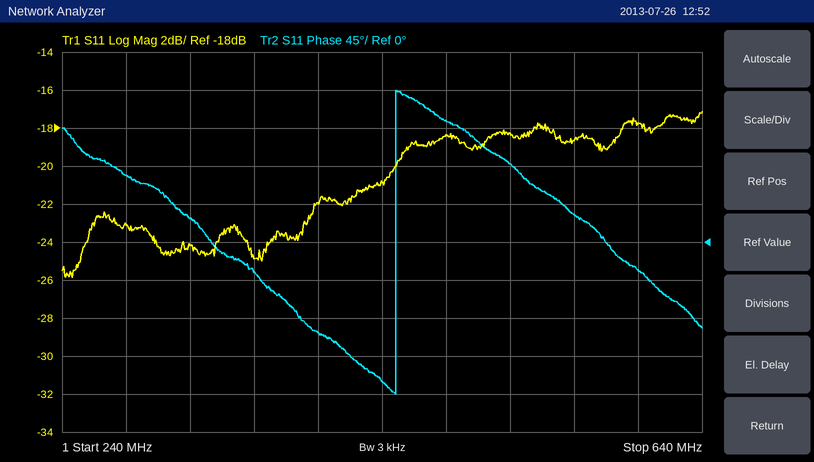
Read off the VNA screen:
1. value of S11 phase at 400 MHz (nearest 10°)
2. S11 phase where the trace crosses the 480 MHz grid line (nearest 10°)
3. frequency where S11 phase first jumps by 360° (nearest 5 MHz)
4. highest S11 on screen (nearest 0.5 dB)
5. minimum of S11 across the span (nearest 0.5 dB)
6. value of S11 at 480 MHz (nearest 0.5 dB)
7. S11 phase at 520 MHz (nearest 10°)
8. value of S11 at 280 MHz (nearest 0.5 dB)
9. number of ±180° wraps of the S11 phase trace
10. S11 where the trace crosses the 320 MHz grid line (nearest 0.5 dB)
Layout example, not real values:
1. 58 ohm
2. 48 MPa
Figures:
1. -110°
2. 140°
3. 450 MHz
4. -17.0 dB
5. -26.0 dB
6. -18.5 dB
7. 90°
8. -23.0 dB
9. 1
10. -24.0 dB
